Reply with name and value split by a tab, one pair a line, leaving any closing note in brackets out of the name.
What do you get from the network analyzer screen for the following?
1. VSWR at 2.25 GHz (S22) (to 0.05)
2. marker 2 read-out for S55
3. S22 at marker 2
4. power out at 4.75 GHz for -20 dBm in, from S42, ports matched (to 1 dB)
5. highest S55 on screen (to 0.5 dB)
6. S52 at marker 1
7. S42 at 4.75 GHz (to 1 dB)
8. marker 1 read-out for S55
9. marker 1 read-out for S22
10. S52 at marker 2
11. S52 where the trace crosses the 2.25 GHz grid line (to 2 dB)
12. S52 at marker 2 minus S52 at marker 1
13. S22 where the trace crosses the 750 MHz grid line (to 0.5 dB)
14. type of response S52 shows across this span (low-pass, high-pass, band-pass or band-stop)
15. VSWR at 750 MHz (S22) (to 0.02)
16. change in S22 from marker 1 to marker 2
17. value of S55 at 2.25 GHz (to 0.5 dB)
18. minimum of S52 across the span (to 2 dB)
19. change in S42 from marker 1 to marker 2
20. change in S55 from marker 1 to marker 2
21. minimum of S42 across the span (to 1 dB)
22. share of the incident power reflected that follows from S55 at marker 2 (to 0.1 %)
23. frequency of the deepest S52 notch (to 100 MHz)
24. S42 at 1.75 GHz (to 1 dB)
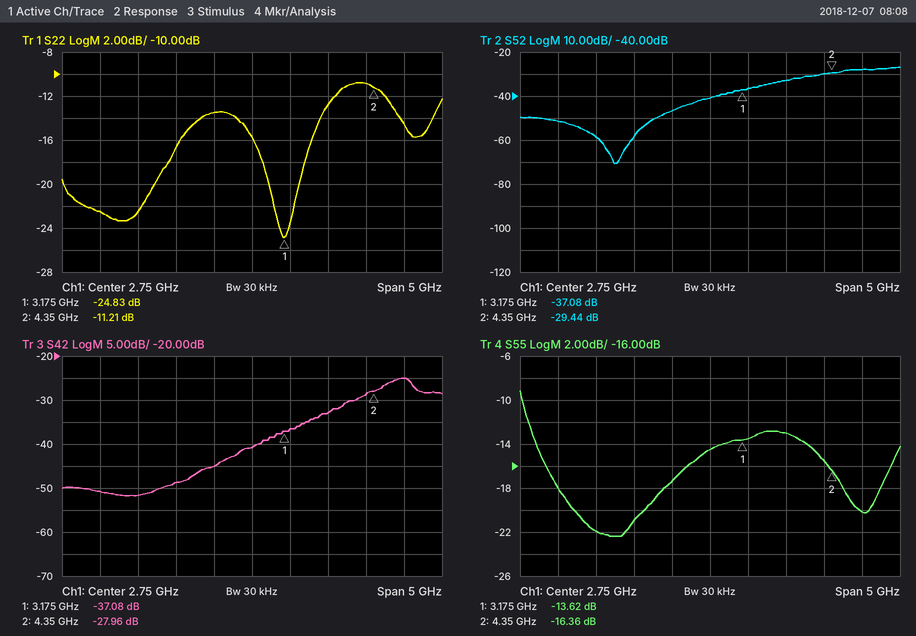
VSWR at 2.25 GHz (S22)	1.55
marker 2 read-out for S55	-16.36 dB
S22 at marker 2	-11.21 dB
power out at 4.75 GHz for -20 dBm in, from S42, ports matched	-45 dBm
highest S55 on screen	-9.0 dB
S52 at marker 1	-37.08 dB
S42 at 4.75 GHz	-25 dB
marker 1 read-out for S55	-13.62 dB
marker 1 read-out for S22	-24.83 dB
S52 at marker 2	-29.44 dB
S52 where the trace crosses the 2.25 GHz grid line	-46 dB
S52 at marker 2 minus S52 at marker 1	7.64 dB
S22 where the trace crosses the 750 MHz grid line	-22.5 dB
type of response S52 shows across this span	high-pass
VSWR at 750 MHz (S22)	1.16
change in S22 from marker 1 to marker 2	13.62 dB
value of S55 at 2.25 GHz	-17.5 dB
minimum of S52 across the span	-70 dB
change in S42 from marker 1 to marker 2	9.12 dB
change in S55 from marker 1 to marker 2	-2.74 dB
minimum of S42 across the span	-52 dB
share of the incident power reflected that follows from S55 at marker 2	2.3 %
frequency of the deepest S52 notch	1.5 GHz
S42 at 1.75 GHz	-49 dB
